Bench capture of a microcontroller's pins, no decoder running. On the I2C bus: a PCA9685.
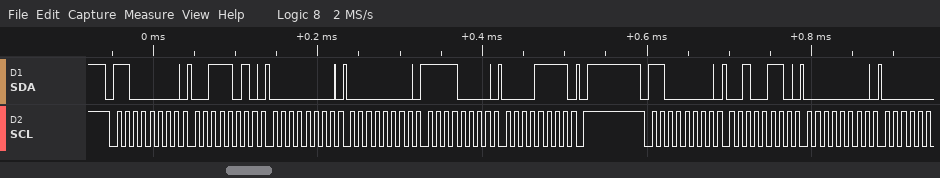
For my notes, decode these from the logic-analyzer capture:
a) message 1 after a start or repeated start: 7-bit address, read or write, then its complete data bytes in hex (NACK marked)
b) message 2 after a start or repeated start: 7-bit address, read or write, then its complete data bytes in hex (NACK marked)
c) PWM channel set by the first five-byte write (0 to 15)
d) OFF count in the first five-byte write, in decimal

0x60 write: 3A 00 00 F0 0F
0x60 write: 26 00
13
4080
